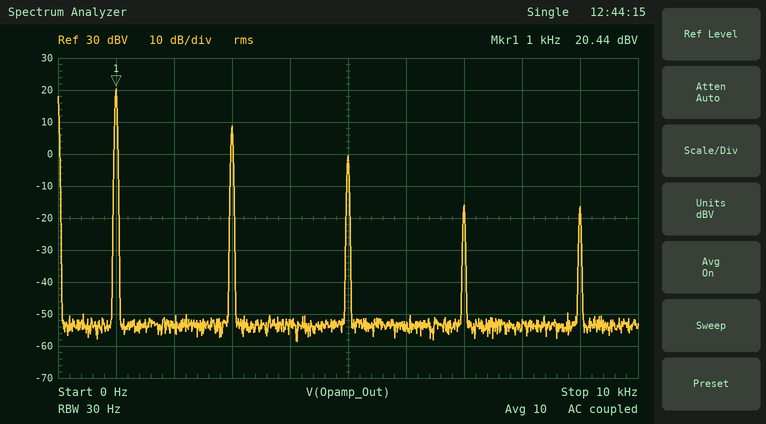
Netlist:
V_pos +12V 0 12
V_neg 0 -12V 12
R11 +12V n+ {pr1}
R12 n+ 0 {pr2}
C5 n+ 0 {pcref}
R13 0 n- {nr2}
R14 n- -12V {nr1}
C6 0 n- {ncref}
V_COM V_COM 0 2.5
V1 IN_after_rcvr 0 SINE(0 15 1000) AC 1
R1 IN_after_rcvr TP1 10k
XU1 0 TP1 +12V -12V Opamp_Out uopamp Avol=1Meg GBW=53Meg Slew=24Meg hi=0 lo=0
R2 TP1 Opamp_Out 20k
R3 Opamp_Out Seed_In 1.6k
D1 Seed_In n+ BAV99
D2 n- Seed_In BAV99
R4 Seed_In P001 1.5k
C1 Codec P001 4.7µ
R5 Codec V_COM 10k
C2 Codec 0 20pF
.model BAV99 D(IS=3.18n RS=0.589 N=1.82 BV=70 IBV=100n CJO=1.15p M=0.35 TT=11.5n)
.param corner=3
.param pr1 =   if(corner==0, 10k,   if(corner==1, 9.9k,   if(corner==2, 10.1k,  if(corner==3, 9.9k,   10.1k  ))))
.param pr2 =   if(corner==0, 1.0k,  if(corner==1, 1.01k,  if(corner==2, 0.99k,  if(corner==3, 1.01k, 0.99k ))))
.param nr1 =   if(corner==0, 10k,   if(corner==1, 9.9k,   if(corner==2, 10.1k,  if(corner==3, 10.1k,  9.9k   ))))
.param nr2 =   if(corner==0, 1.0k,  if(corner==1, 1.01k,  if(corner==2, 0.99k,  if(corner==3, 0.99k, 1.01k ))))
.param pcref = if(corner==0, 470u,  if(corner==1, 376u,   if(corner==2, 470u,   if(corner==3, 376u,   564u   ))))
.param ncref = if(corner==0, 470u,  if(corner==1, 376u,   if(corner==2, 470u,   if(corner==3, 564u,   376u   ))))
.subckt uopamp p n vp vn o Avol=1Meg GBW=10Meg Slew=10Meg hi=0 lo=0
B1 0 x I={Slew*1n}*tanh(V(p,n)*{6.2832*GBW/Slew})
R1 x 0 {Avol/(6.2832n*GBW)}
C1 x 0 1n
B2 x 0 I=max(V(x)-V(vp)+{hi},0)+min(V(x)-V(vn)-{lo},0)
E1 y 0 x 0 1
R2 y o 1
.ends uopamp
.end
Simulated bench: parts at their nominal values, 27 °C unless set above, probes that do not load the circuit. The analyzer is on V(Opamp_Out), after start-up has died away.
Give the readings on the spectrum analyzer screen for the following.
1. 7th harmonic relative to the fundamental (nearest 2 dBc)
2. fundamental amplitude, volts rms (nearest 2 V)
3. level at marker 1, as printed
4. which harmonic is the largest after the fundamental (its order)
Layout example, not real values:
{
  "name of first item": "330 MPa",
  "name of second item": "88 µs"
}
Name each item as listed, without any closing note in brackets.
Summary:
{
  "7th harmonic relative to the fundamental": "-36 dBc",
  "fundamental amplitude, volts rms": "10 V",
  "level at marker 1, as printed": "20.44 dBV",
  "which harmonic is the largest after the fundamental": "3"
}
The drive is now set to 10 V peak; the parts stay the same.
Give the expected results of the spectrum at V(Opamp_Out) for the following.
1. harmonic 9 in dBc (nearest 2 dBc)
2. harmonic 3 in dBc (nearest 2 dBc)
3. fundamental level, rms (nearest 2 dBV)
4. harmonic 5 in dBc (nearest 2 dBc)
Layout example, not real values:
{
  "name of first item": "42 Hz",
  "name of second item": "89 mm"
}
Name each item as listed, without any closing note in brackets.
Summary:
{
  "harmonic 9 in dBc": "-40 dBc",
  "harmonic 3 in dBc": "-14 dBc",
  "fundamental level, rms": "20 dBV",
  "harmonic 5 in dBc": "-48 dBc"
}
